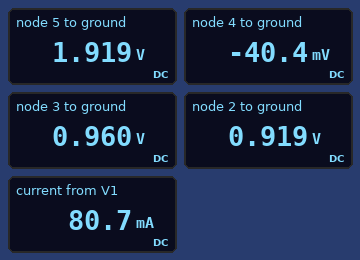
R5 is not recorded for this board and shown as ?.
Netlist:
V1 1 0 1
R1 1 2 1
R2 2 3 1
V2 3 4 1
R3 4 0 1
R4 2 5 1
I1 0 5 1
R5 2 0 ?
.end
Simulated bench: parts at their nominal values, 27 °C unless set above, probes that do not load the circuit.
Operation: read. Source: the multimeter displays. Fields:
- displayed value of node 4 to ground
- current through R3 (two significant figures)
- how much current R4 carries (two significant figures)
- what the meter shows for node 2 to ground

-40.4 mV
40 mA
1.0 A
0.919 V
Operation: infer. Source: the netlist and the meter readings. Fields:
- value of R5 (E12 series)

0.82 Ω
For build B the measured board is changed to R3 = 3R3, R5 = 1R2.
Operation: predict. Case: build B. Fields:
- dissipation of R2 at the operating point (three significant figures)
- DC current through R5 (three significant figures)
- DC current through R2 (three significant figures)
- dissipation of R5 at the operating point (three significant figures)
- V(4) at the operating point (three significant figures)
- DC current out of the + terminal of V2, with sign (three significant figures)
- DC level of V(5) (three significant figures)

352 µW
901 mA
18.8 mA
973 mW
61.9 mV
-18.8 mA
2.08 V
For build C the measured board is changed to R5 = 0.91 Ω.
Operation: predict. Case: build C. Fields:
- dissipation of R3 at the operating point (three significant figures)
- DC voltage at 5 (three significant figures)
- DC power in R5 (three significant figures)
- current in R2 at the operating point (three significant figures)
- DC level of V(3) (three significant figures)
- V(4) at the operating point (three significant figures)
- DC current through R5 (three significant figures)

362 µW
1.96 V
1.02 W
19.0 mA
981 mV
-19.0 mV
1.06 A
